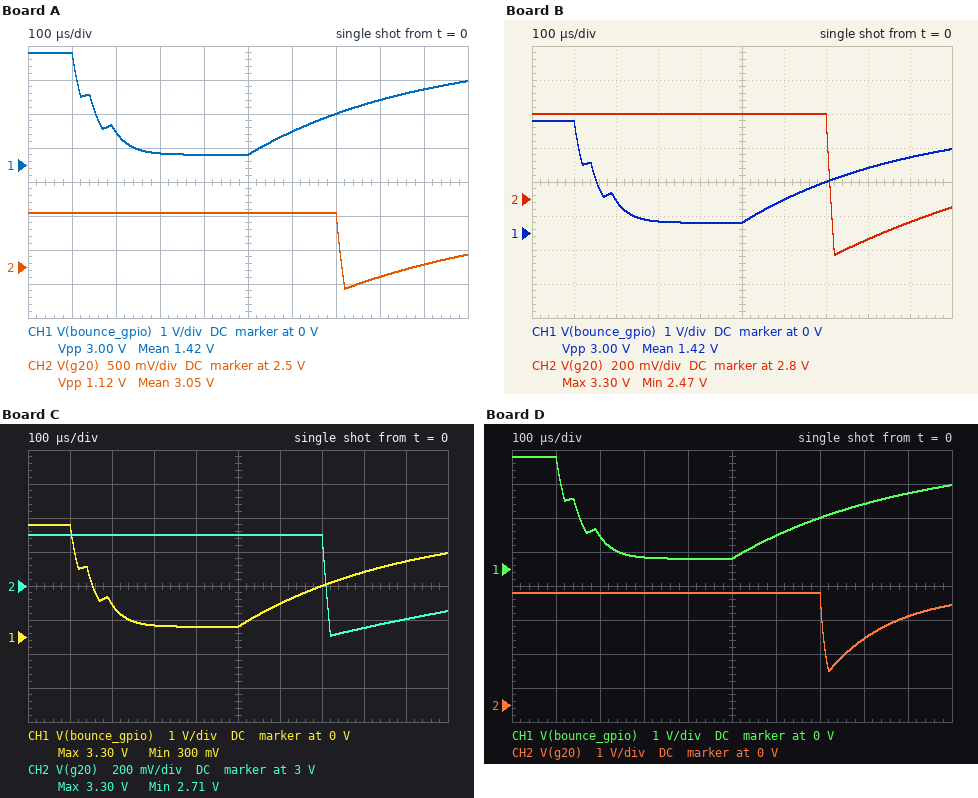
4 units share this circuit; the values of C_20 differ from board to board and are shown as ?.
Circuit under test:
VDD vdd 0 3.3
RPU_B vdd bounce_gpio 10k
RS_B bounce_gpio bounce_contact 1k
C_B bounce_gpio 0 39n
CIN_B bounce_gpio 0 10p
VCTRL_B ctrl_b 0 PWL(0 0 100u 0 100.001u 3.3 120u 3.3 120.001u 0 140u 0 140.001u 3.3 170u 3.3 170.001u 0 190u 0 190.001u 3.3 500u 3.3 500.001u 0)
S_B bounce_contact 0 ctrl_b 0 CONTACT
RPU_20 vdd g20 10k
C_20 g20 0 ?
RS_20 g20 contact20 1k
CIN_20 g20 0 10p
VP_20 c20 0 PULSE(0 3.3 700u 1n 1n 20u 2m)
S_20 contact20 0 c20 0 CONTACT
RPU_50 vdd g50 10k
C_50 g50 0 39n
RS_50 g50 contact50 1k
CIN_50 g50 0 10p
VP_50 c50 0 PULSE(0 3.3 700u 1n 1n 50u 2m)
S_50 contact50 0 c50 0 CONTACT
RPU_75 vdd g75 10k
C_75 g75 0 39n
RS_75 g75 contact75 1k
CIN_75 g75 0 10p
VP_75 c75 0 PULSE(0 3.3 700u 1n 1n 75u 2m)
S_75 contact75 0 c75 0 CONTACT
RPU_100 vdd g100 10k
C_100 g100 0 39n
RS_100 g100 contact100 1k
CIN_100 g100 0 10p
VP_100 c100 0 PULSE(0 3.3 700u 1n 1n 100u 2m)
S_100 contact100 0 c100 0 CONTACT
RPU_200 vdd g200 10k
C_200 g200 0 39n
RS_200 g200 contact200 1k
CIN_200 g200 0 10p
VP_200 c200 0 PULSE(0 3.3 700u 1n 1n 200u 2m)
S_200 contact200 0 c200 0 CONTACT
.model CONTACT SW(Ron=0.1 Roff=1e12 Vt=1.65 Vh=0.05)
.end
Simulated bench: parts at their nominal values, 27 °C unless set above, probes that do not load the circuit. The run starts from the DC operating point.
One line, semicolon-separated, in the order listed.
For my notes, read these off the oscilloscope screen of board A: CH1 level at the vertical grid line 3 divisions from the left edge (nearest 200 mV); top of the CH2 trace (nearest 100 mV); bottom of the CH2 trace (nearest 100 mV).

400 mV; 3.3 V; 2.2 V
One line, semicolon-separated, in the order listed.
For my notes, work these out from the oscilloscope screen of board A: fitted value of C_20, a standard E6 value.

47 nF
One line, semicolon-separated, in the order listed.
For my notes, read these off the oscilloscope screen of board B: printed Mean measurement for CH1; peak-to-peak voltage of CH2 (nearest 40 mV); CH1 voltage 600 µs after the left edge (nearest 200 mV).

1.42 V; 840 mV; 1.0 V
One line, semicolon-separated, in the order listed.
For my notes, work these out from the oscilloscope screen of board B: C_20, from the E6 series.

68 nF
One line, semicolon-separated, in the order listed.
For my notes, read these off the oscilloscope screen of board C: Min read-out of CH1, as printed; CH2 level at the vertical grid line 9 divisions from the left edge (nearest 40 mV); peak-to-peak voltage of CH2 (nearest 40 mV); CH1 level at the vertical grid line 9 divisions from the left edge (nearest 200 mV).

300 mV; 2.80 V; 600 mV; 2.2 V
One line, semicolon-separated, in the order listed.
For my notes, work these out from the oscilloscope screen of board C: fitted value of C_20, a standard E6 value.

100 nF
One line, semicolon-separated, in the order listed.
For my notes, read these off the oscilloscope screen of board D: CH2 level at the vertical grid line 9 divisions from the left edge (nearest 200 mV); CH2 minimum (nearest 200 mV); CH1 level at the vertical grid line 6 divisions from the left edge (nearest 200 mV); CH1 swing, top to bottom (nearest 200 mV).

2.6 V; 1.0 V; 1.0 V; 3.0 V
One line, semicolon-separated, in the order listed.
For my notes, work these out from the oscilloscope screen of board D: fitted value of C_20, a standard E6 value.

15 nF
